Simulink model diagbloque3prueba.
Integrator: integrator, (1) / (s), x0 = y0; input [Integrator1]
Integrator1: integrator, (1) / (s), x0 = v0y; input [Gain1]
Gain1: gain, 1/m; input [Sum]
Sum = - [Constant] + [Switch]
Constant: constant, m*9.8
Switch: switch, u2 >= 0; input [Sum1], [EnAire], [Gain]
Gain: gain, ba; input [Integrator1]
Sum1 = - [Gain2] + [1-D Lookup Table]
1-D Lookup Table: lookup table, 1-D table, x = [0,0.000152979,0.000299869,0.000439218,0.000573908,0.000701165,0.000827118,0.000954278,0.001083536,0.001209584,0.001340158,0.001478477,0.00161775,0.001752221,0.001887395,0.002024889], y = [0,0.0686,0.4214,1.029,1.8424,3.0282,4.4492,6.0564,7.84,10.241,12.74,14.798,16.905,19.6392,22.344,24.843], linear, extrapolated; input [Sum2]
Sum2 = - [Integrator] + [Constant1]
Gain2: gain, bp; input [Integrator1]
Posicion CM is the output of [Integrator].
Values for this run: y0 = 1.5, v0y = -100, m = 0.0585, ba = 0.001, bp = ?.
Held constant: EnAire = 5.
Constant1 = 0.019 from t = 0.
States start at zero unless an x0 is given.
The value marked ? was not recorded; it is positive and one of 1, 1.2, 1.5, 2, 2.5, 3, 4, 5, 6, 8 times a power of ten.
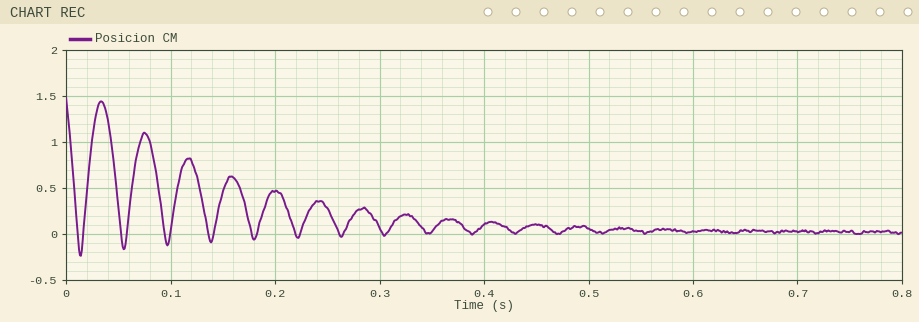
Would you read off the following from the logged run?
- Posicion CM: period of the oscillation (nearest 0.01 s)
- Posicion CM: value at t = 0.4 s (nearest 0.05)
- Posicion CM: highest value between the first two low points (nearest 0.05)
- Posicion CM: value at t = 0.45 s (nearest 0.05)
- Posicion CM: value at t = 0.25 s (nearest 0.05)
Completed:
0.04 s
0.10
1.45
0.10
0.30
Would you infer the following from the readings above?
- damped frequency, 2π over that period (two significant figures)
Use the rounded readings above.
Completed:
160 rad/s
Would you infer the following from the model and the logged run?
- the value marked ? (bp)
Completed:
0.8
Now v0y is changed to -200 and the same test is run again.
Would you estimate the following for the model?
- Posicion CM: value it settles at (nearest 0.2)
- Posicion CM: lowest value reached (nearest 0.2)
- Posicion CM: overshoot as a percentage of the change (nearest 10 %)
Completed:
0.0
-0.4
30 %
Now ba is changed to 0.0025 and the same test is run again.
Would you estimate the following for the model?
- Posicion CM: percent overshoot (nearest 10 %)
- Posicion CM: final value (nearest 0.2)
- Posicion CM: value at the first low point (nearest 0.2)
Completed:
20 %
0.0
-0.2
